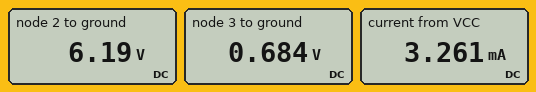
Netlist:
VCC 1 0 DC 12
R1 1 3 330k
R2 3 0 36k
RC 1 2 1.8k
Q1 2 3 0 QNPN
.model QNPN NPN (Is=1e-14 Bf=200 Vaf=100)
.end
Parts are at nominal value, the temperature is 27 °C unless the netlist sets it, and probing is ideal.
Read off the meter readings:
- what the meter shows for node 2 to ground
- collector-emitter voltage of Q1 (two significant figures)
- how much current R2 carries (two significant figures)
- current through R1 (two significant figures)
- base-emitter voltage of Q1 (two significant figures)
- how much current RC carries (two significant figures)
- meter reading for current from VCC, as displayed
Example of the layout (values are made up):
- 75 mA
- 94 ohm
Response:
- 6.19 V
- 6.2 V
- 19 µA
- 34 µA
- 680 mV
- 3.2 mA
- 3.261 mA
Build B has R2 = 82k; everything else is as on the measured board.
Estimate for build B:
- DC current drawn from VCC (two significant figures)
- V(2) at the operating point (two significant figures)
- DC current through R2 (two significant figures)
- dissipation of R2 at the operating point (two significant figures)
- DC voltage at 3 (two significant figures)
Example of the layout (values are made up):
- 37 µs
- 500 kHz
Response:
- 5.3 mA
- 2.6 V
- 8.5 µA
- 5.9 µW
- 700 mV
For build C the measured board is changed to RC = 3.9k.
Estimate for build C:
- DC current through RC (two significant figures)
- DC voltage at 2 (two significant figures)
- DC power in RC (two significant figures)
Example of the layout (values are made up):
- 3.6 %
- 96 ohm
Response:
- 3.0 mA
- 250 mV
- 35 mW
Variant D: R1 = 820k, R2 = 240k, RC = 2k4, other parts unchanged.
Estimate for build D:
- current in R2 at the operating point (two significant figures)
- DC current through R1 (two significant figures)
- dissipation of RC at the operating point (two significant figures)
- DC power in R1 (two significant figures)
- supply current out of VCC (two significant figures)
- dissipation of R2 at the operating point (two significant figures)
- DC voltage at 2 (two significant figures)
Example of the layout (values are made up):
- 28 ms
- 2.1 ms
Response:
- 2.8 µA
- 14 µA
- 13 mW
- 160 µW
- 2.3 mA
- 1.9 µW
- 6.4 V
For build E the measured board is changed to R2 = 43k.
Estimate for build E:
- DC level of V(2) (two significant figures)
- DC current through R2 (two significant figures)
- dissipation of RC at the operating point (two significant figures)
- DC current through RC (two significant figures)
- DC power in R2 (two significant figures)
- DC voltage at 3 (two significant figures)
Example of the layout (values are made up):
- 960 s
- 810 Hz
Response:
- 5.1 V
- 16 µA
- 26 mW
- 3.8 mA
- 11 µW
- 690 mV
